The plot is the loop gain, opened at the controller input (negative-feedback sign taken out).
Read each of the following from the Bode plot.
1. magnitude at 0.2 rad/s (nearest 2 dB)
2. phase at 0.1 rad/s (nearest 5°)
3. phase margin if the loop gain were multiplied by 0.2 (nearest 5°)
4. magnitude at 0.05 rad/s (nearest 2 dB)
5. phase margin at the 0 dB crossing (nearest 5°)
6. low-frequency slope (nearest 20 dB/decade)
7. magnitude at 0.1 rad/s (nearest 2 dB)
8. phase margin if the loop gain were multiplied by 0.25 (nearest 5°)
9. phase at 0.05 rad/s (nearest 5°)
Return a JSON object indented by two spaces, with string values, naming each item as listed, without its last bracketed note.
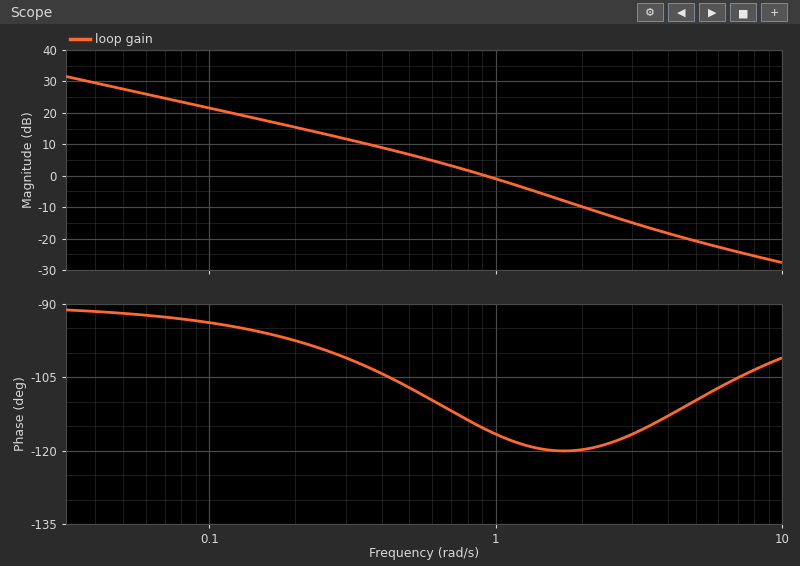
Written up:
{
  "magnitude at 0.2 rad/s": "16 dB",
  "phase at 0.1 rad/s": "-95°",
  "phase margin if the loop gain were multiplied by 0.2": "80°",
  "magnitude at 0.05 rad/s": "28 dB",
  "phase margin at the 0 dB crossing": "65°",
  "low-frequency slope": "-20 dB/decade",
  "magnitude at 0.1 rad/s": "22 dB",
  "phase margin if the loop gain were multiplied by 0.25": "80°",
  "phase at 0.05 rad/s": "-90°"
}
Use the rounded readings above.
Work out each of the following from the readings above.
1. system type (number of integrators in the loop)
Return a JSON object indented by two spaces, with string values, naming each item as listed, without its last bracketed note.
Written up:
{
  "system type": "1"
}
